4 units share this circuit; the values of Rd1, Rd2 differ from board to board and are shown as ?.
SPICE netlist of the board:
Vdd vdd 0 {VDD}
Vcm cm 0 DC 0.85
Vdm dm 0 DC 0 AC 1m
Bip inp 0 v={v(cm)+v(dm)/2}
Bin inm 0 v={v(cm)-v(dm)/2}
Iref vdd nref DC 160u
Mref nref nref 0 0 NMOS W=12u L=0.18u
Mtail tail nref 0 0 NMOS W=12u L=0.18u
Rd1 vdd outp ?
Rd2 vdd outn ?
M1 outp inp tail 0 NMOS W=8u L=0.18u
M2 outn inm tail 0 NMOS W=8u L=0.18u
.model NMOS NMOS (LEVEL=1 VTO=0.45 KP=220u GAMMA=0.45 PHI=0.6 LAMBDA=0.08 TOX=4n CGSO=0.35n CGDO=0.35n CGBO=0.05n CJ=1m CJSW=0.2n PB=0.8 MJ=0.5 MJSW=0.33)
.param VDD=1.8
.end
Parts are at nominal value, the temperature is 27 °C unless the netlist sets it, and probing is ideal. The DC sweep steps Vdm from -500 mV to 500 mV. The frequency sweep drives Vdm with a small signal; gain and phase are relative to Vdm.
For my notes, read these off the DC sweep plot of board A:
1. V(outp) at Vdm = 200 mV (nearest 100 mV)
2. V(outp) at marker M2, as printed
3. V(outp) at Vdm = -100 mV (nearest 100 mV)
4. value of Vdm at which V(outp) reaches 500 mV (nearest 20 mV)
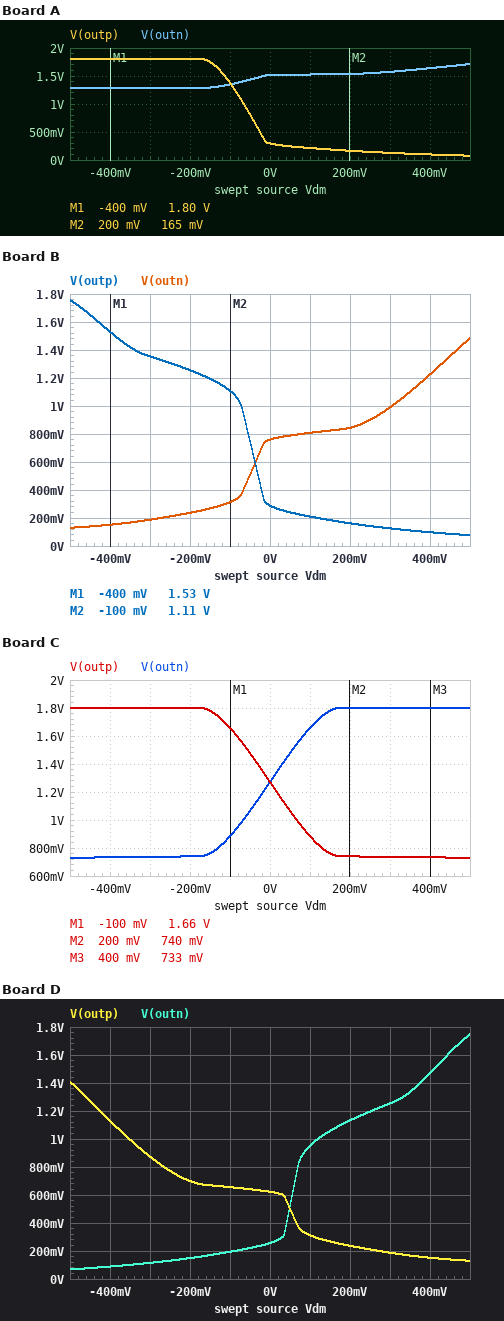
200 mV
165 mV
1.4 V
-20 mV
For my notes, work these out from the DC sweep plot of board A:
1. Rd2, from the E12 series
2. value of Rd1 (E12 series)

3.3 kΩ
22 kΩ
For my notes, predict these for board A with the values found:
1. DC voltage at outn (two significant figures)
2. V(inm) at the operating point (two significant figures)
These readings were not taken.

1.5 V
850 mV
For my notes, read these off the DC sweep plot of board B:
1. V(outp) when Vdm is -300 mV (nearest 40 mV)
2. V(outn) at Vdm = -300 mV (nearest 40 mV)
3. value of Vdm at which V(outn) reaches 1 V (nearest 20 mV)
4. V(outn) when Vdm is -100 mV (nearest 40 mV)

1.36 V
200 mV
300 mV
320 mV
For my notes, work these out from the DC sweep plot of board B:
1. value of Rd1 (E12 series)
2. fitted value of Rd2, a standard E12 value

22 kΩ
12 kΩ
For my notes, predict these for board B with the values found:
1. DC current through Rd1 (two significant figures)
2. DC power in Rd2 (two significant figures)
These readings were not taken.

69 µA
90 µW
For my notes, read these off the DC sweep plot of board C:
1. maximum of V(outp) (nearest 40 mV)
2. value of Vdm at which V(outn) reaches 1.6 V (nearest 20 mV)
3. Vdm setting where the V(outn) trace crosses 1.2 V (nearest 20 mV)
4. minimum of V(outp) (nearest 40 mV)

1.80 V
80 mV
-20 mV
720 mV
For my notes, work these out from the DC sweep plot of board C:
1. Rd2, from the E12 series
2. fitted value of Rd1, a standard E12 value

6.8 kΩ
6.8 kΩ
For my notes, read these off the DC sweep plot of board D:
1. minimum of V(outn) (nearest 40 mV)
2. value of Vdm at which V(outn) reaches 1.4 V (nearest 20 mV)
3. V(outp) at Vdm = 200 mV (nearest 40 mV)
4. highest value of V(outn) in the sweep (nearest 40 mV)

80 mV
380 mV
240 mV
1.76 V
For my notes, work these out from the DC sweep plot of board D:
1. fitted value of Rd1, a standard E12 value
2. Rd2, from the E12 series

12 kΩ
27 kΩ
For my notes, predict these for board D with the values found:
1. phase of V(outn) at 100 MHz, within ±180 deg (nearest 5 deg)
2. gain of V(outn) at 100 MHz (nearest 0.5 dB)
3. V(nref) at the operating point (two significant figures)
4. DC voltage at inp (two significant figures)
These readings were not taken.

0 deg
-1.0 dB
590 mV
850 mV
